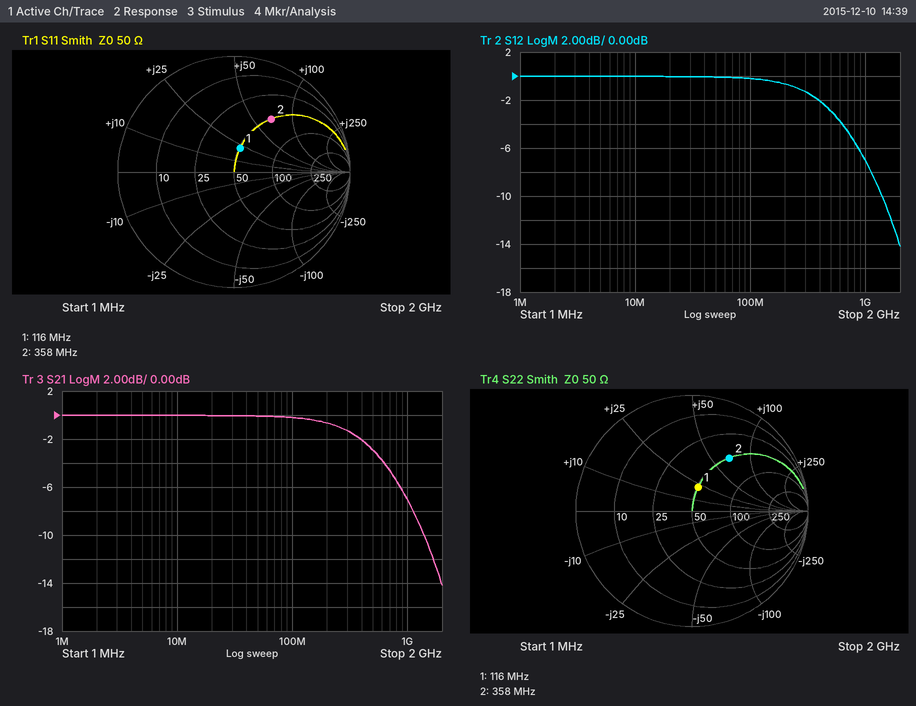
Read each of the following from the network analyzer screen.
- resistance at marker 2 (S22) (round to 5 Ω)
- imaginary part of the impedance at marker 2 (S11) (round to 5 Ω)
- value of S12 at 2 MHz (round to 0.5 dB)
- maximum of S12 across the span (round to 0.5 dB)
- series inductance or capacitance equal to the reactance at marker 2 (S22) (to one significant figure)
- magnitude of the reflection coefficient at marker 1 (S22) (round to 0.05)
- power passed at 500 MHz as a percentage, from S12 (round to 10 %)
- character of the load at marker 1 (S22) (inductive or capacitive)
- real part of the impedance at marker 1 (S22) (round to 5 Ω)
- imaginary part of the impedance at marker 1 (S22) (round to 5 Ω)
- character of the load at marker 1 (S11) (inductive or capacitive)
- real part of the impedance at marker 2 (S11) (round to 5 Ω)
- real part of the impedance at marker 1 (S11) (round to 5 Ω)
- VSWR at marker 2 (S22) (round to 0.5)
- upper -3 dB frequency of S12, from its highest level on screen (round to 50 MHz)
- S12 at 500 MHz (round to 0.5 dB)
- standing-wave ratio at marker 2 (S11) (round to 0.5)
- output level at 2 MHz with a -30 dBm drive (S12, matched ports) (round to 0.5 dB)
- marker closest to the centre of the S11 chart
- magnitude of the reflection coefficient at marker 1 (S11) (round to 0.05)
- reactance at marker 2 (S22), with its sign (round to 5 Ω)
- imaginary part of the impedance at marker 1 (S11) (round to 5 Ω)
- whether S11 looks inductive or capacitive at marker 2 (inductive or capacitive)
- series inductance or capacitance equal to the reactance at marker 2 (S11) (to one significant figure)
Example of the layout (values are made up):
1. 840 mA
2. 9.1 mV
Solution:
1. 50 Ω
2. +70 Ω
3. 0.0 dB
4. 0.0 dB
5. 30 nH
6. 0.20
7. 50 %
8. inductive
9. 50 Ω
10. +20 Ω
11. inductive
12. 50 Ω
13. 50 Ω
14. 3.5
15. 500 MHz
16. -3.0 dB
17. 3.5
18. -30.0 dBm
19. marker 1
20. 0.20
21. +70 Ω
22. +20 Ω
23. inductive
24. 30 nH
